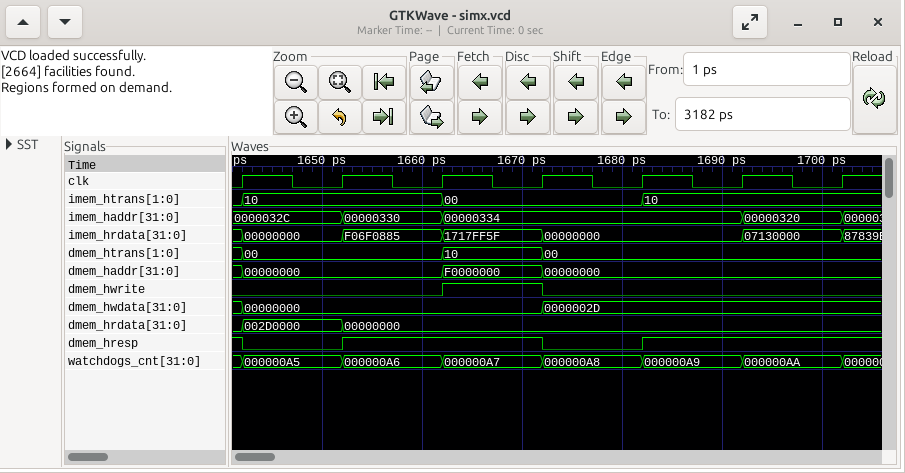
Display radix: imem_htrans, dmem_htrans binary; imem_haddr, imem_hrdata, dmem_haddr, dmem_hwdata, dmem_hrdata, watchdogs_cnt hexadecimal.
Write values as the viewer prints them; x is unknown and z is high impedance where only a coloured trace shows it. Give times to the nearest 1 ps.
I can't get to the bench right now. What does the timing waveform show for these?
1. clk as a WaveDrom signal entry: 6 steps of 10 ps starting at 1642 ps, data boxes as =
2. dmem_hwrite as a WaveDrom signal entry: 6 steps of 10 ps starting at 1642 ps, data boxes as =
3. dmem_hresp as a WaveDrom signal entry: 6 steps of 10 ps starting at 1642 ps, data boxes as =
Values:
{name: 'clk', wave: 'p.....'}
{name: 'dmem_hwrite', wave: '0.10..'}
{name: 'dmem_hresp', wave: '01.01.'}
